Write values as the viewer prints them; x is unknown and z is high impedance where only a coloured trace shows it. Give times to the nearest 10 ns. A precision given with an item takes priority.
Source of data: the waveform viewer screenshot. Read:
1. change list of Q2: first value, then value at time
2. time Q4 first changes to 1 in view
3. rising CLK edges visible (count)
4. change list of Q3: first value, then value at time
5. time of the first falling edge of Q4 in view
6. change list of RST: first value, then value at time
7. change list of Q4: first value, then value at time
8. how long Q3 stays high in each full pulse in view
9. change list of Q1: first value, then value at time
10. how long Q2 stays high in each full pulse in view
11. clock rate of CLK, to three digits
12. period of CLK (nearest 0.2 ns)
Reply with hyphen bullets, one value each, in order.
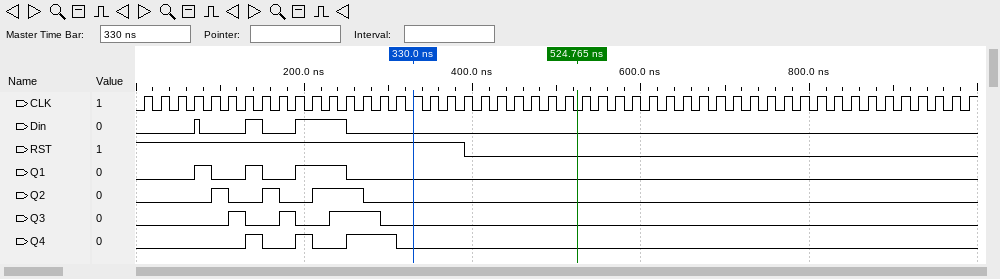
- 0, 1 at 90 ns, 0 at 110 ns, 1 at 150 ns, 0 at 170 ns, 1 at 210 ns, 0 at 270 ns
- 130 ns
- 50
- 0, 1 at 110 ns, 0 at 130 ns, 1 at 170 ns, 0 at 190 ns, 1 at 230 ns, 0 at 290 ns
- 150 ns
- 1, 0 at 390 ns
- 0, 1 at 130 ns, 0 at 150 ns, 1 at 190 ns, 0 at 210 ns, 1 at 250 ns, 0 at 310 ns
- 20 ns, 20 ns, 60 ns
- 0, 1 at 70 ns, 0 at 90 ns, 1 at 130 ns, 0 at 150 ns, 1 at 190 ns, 0 at 250 ns
- 20 ns, 20 ns, 60 ns
- 50.0 MHz
- 20 ns
